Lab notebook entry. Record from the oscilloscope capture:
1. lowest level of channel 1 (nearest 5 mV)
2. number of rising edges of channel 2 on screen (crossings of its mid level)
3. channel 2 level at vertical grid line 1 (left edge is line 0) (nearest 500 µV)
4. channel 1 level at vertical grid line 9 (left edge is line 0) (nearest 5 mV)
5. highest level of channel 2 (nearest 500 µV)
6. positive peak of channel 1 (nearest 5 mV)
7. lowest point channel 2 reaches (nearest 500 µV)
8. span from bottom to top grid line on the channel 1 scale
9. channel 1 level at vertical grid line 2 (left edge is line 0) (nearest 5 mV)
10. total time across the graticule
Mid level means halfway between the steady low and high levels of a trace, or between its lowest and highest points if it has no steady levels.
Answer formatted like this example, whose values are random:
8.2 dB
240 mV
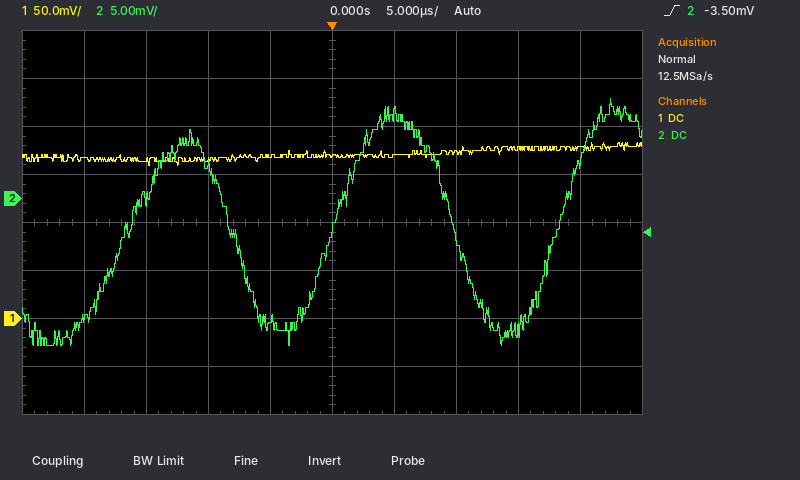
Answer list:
160 mV
3
-12.5 mV
180 mV
10.5 mV
185 mV
-15.5 mV
400 mV
165 mV
50 µs
